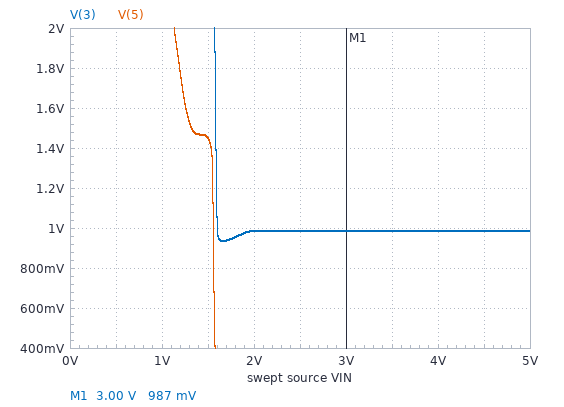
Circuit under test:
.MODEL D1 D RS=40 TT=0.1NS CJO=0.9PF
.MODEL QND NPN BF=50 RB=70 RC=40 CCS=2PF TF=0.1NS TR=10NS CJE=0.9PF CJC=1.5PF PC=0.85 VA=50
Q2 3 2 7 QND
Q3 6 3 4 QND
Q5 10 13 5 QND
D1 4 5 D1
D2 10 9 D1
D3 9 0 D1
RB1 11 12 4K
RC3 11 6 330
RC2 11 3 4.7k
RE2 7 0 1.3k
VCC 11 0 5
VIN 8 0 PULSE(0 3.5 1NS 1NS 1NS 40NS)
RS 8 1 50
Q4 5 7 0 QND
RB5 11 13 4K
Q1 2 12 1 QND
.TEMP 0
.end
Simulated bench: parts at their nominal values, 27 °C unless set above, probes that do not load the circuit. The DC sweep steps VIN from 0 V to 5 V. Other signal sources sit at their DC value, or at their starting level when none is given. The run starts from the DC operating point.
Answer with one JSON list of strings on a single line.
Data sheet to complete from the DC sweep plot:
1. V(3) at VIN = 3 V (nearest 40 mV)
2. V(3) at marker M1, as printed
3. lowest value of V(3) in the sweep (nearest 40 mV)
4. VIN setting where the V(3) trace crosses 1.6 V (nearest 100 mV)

["1.00 V", "987 mV", "920 mV", "1.6 V"]
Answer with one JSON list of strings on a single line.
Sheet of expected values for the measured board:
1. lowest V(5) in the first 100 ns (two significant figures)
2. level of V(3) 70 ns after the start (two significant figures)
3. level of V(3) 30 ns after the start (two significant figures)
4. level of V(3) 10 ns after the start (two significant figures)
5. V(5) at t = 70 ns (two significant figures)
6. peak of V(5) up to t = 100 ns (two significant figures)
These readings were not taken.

["-43 mV", "3.2 V", "990 mV", "1.1 V", "1.7 V", "3.6 V"]
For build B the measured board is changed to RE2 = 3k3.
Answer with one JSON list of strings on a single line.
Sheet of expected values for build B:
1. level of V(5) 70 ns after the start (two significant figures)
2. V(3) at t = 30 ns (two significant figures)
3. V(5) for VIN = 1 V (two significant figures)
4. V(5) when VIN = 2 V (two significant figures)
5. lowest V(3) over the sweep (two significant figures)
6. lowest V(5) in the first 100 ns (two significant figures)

["1.6 V", "1.0 V", "3.0 V", "64 mV", "970 mV", "-11 mV"]
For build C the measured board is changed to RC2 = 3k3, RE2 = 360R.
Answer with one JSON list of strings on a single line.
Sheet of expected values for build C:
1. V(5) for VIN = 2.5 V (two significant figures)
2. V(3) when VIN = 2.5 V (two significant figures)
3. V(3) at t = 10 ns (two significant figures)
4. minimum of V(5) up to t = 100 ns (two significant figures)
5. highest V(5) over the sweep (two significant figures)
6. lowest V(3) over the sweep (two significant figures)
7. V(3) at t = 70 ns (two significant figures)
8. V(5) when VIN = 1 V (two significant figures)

["99 mV", "900 mV", "950 mV", "-120 mV", "3.4 V", "640 mV", "3.9 V", "1.5 V"]
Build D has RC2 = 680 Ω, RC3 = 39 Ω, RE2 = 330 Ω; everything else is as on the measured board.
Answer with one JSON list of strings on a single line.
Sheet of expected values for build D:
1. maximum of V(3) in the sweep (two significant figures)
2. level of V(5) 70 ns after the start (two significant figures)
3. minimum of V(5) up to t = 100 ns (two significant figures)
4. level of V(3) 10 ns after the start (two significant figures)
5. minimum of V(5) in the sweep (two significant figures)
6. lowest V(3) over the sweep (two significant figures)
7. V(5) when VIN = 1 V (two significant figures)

["5.0 V", "3.5 V", "13 mV", "1.4 V", "61 mV", "1.3 V", "3.0 V"]
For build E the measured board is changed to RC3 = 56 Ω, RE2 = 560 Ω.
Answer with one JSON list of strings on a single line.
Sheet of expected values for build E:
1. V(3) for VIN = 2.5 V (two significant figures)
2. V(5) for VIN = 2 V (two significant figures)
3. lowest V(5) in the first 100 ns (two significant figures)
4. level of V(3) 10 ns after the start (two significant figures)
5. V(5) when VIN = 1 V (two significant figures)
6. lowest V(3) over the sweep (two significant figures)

["920 mV", "75 mV", "-210 mV", "970 mV", "1.5 V", "660 mV"]
